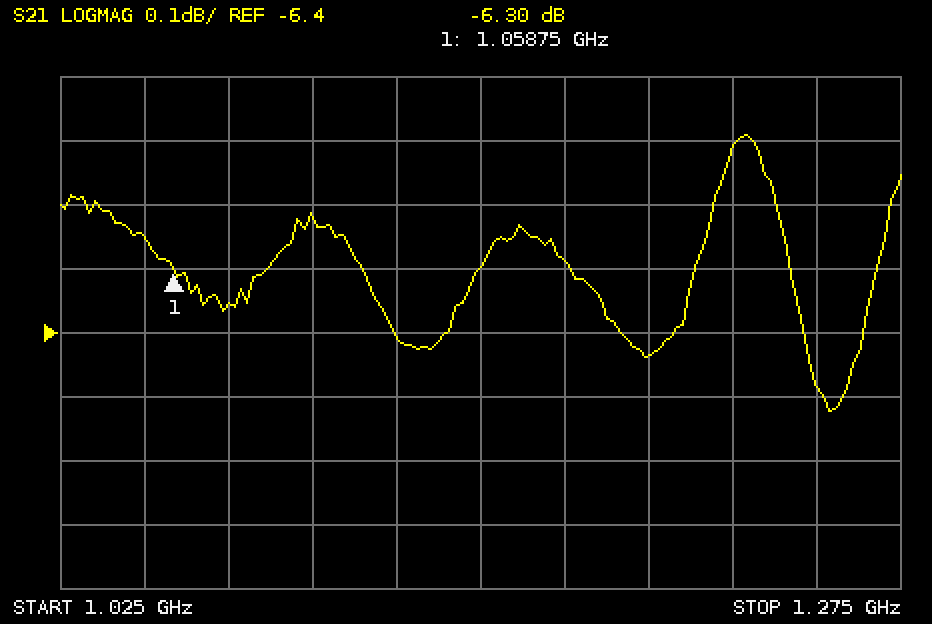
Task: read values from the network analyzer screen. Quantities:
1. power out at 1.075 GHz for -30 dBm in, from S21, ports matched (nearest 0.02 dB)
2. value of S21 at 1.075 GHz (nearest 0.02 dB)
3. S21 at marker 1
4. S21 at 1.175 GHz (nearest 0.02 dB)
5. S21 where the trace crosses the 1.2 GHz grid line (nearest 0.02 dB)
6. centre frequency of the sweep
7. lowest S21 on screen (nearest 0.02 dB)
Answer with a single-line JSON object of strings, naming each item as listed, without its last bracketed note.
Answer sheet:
{"power out at 1.075 GHz for -30 dBm in, from S21, ports matched": "-36.36 dBm", "value of S21 at 1.075 GHz": "-6.36 dB", "S21 at marker 1": "-6.30 dB", "S21 at 1.175 GHz": "-6.28 dB", "S21 where the trace crosses the 1.2 GHz grid line": "-6.44 dB", "centre frequency of the sweep": "1.15 GHz", "lowest S21 on screen": "-6.52 dB"}
